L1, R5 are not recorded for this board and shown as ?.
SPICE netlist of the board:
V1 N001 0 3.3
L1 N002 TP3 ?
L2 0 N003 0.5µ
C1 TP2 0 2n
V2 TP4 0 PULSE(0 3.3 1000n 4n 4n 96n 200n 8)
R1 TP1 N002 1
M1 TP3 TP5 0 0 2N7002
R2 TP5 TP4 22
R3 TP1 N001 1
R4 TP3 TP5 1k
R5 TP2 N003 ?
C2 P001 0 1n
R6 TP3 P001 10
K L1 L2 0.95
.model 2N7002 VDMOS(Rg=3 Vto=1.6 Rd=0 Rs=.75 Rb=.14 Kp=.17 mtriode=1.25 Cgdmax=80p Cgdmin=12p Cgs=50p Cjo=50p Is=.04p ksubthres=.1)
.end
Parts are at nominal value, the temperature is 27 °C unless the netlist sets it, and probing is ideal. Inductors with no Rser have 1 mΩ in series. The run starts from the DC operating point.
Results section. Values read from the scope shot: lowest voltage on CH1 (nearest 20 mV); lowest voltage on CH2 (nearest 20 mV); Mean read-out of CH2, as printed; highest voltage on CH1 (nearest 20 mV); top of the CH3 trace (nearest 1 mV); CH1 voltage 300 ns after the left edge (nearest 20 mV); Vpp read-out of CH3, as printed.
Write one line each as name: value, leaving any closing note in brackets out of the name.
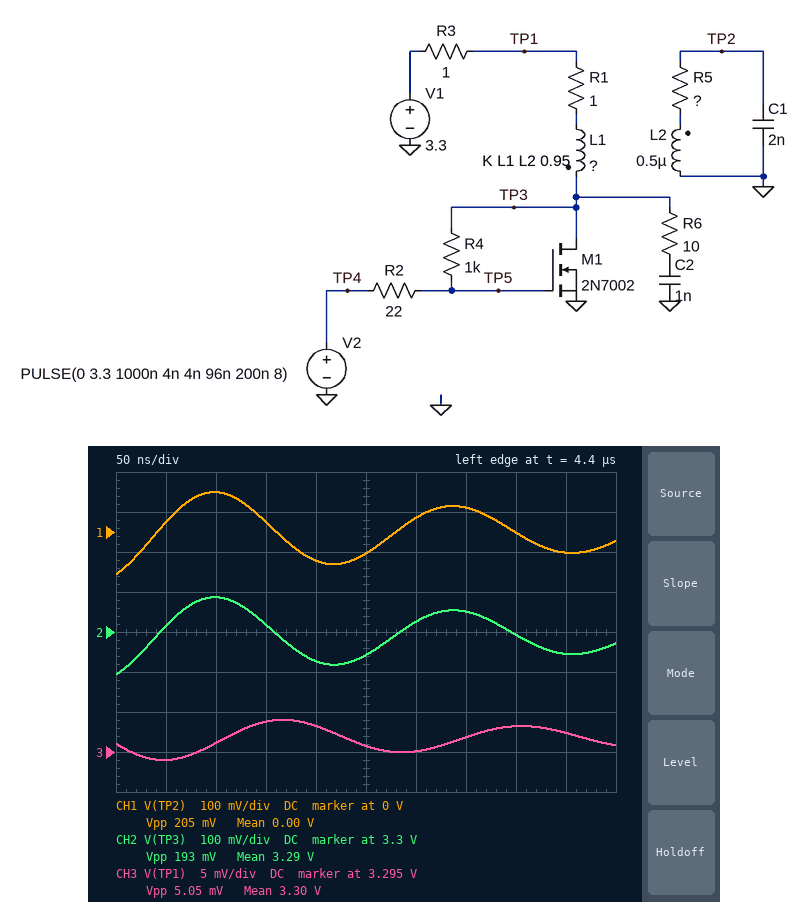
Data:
lowest voltage on CH1: -100 mV
lowest voltage on CH2: 3.20 V
Mean read-out of CH2, as printed: 3.29 V
highest voltage on CH1: 100 mV
top of the CH3 trace: 3.299 V
CH1 voltage 300 ns after the left edge: 40 mV
Vpp read-out of CH3, as printed: 5.05 mV
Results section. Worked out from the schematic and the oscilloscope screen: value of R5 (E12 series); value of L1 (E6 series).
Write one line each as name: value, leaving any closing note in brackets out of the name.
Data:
value of R5: 0.82 Ω
value of L1: 470 nH
